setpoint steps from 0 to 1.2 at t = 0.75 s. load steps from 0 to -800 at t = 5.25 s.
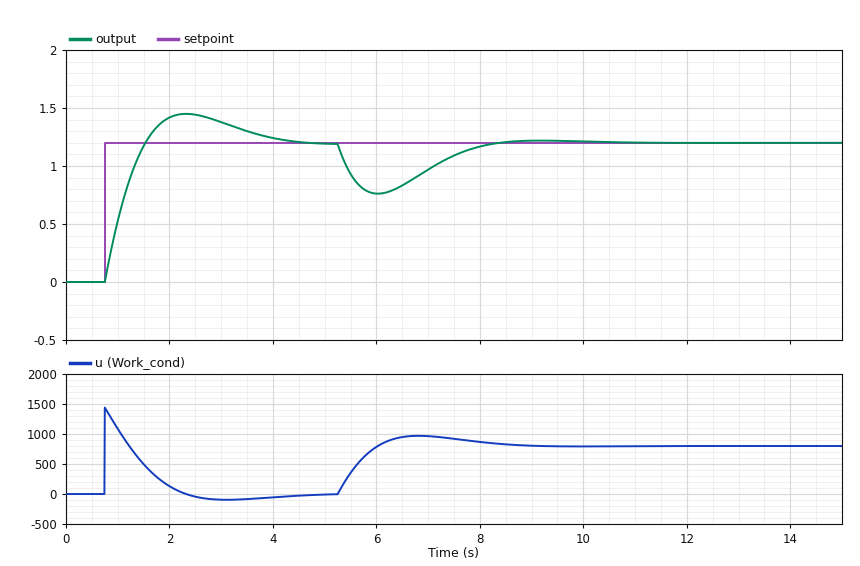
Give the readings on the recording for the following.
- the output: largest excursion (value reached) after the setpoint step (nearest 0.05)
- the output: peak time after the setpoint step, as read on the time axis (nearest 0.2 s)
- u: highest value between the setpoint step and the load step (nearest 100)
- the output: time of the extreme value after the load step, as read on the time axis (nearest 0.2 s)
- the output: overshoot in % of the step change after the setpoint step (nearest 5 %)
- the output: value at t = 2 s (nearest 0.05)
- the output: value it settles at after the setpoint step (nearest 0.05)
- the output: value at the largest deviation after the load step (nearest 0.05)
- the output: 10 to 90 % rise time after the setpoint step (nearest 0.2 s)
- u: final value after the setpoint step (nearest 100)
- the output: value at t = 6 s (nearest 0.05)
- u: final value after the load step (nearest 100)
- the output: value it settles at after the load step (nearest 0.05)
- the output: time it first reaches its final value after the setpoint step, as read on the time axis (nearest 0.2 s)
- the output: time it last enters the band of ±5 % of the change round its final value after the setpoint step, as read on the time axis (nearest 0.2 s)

1.45
2.4 s
1400
6.0 s
20 %
1.40
1.20
0.75
0.6 s
0
0.75
800
1.20
1.6 s
3.8 s
